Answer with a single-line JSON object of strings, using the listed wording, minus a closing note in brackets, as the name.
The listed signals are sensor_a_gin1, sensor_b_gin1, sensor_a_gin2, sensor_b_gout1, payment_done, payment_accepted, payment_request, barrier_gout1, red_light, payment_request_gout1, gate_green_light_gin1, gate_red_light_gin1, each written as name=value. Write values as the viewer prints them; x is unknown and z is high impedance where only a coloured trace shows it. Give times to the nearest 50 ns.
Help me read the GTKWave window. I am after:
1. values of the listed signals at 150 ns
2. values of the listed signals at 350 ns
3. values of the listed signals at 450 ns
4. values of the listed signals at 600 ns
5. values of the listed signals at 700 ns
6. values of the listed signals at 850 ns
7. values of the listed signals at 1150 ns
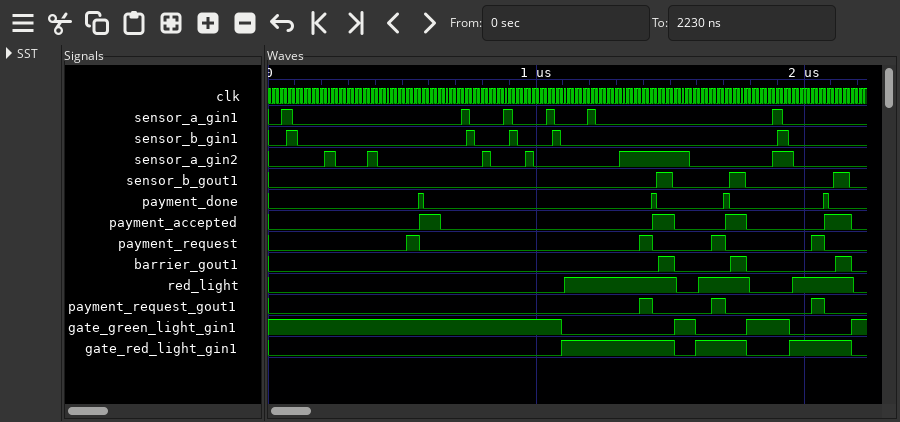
{"values of the listed signals at 150 ns": "sensor_a_gin1=0, sensor_b_gin1=0, sensor_a_gin2=0, sensor_b_gout1=0, payment_done=0, payment_accepted=0, payment_request=0, barrier_gout1=0, red_light=0, payment_request_gout1=0, gate_green_light_gin1=1, gate_red_light_gin1=0", "values of the listed signals at 350 ns": "sensor_a_gin1=0, sensor_b_gin1=0, sensor_a_gin2=0, sensor_b_gout1=0, payment_done=0, payment_accepted=0, payment_request=0, barrier_gout1=0, red_light=0, payment_request_gout1=0, gate_green_light_gin1=1, gate_red_light_gin1=0", "values of the listed signals at 450 ns": "sensor_a_gin1=0, sensor_b_gin1=0, sensor_a_gin2=0, sensor_b_gout1=0, payment_done=0, payment_accepted=0, payment_request=0, barrier_gout1=0, red_light=0, payment_request_gout1=0, gate_green_light_gin1=1, gate_red_light_gin1=0", "values of the listed signals at 600 ns": "sensor_a_gin1=0, sensor_b_gin1=0, sensor_a_gin2=0, sensor_b_gout1=0, payment_done=0, payment_accepted=1, payment_request=0, barrier_gout1=0, red_light=0, payment_request_gout1=0, gate_green_light_gin1=1, gate_red_light_gin1=0", "values of the listed signals at 700 ns": "sensor_a_gin1=0, sensor_b_gin1=0, sensor_a_gin2=0, sensor_b_gout1=0, payment_done=0, payment_accepted=0, payment_request=0, barrier_gout1=0, red_light=0, payment_request_gout1=0, gate_green_light_gin1=1, gate_red_light_gin1=0", "values of the listed signals at 850 ns": "sensor_a_gin1=0, sensor_b_gin1=0, sensor_a_gin2=0, sensor_b_gout1=0, payment_done=0, payment_accepted=0, payment_request=0, barrier_gout1=0, red_light=0, payment_request_gout1=0, gate_green_light_gin1=1, gate_red_light_gin1=0", "values of the listed signals at 1150 ns": "sensor_a_gin1=0, sensor_b_gin1=0, sensor_a_gin2=0, sensor_b_gout1=0, payment_done=0, payment_accepted=0, payment_request=0, barrier_gout1=0, red_light=1, payment_request_gout1=0, gate_green_light_gin1=0, gate_red_light_gin1=1"}
